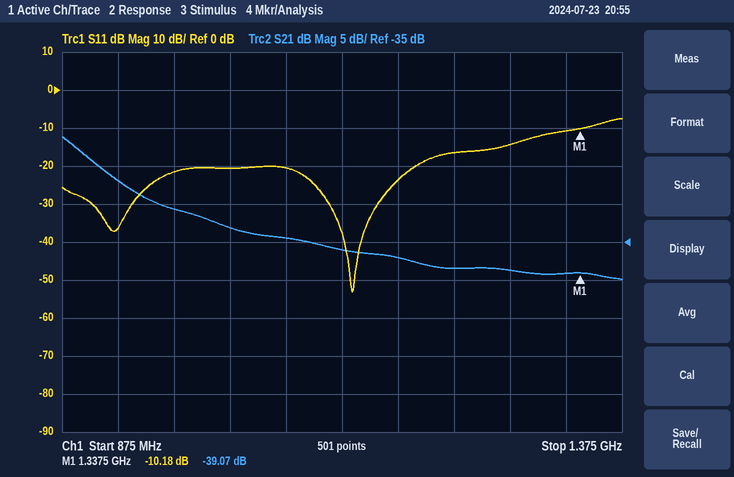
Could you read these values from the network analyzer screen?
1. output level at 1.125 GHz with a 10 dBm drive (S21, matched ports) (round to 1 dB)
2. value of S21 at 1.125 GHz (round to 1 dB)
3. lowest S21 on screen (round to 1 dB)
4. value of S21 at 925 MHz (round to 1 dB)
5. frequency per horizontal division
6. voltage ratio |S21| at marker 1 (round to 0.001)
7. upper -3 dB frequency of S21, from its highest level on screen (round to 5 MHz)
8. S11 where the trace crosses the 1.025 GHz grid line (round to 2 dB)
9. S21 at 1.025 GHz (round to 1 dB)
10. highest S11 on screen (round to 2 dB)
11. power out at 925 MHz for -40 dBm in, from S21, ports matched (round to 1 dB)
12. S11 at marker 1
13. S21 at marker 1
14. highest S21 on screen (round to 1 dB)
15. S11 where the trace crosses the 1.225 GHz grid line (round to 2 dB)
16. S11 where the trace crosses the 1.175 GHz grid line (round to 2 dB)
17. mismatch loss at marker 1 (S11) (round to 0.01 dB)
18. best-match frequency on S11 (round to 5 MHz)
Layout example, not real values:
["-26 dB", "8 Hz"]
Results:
["-26 dBm", "-36 dB", "-40 dB", "-27 dB", "50 MHz", "0.011", "900 MHz", "-20 dB", "-33 dB", "-8 dB", "-67 dBm", "-10.18 dB", "-39.07 dB", "-21 dB", "-16 dB", "-24 dB", "0.44 dB", "1.135 GHz"]
